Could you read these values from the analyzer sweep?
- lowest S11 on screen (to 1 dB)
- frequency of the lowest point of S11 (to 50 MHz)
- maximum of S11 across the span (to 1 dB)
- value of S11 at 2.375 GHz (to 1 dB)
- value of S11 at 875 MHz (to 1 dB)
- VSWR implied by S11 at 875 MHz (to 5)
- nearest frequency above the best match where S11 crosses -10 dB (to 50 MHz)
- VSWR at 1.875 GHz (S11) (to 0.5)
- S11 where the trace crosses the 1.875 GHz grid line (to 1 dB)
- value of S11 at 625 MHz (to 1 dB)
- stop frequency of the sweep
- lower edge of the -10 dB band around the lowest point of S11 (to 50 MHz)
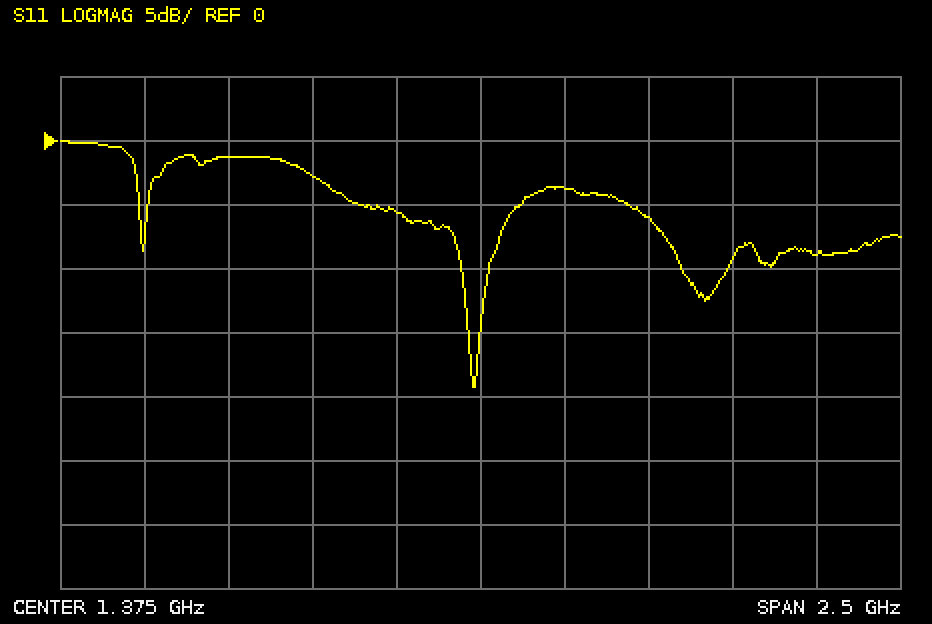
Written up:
-19 dB
1.35 GHz
0 dB
-9 dB
-3 dB
5
1.40 GHz
3.0
-6 dB
-1 dB
2.625 GHz
1.30 GHz
